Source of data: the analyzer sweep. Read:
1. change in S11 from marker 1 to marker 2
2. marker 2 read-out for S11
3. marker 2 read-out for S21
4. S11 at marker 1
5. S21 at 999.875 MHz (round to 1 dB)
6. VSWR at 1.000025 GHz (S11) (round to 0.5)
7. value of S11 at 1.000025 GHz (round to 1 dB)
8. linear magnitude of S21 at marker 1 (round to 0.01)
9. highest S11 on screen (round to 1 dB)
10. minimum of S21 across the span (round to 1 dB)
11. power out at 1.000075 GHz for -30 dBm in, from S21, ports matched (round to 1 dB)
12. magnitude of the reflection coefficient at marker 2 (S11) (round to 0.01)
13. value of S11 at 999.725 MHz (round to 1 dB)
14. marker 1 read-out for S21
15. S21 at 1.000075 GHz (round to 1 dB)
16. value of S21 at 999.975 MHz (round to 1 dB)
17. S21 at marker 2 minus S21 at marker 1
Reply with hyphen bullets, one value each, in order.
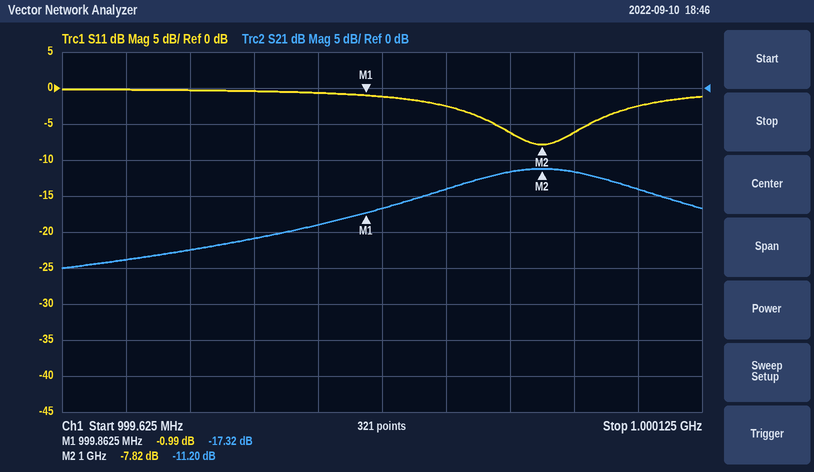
- -6.83 dB
- -7.82 dB
- -11.20 dB
- -0.99 dB
- -17 dB
- 3.0
- -6 dB
- 0.14
- 0 dB
- -25 dB
- -44 dBm
- 0.41
- 0 dB
- -17.32 dB
- -14 dB
- -12 dB
- 6.12 dB
